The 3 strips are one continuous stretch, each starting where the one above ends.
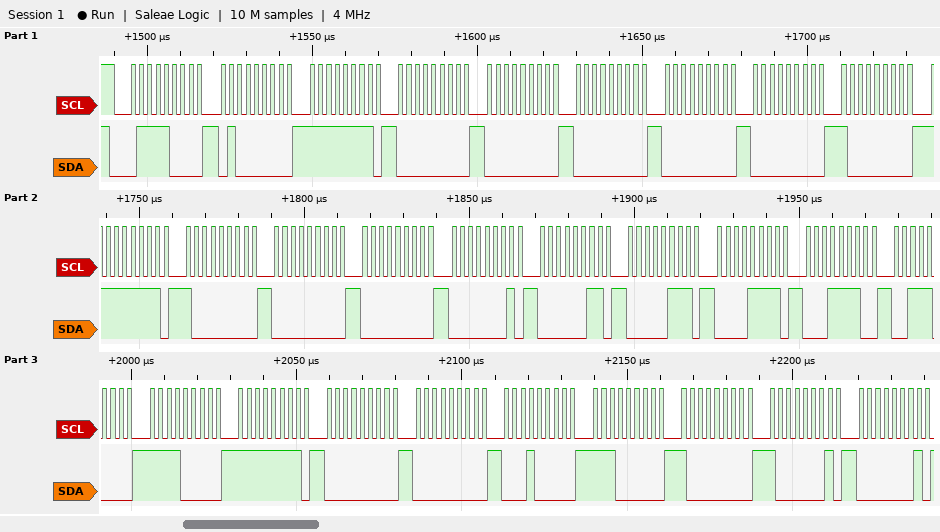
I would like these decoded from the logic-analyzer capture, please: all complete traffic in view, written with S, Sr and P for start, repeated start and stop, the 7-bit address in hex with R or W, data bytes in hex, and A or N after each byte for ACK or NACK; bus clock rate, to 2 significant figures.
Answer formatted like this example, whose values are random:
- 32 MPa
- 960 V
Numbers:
- S 3CW A 40 A FF A 00 A 00 A 00 A 00 A 00 A 80 A FF A 80 A 00 A 00 A 01 A 03 A 07 A 0F A 1E A 38 A F0 A FF A 00 A 00 A 10 A E0 A 80 A 81 A 01 A
- 400 kHz
